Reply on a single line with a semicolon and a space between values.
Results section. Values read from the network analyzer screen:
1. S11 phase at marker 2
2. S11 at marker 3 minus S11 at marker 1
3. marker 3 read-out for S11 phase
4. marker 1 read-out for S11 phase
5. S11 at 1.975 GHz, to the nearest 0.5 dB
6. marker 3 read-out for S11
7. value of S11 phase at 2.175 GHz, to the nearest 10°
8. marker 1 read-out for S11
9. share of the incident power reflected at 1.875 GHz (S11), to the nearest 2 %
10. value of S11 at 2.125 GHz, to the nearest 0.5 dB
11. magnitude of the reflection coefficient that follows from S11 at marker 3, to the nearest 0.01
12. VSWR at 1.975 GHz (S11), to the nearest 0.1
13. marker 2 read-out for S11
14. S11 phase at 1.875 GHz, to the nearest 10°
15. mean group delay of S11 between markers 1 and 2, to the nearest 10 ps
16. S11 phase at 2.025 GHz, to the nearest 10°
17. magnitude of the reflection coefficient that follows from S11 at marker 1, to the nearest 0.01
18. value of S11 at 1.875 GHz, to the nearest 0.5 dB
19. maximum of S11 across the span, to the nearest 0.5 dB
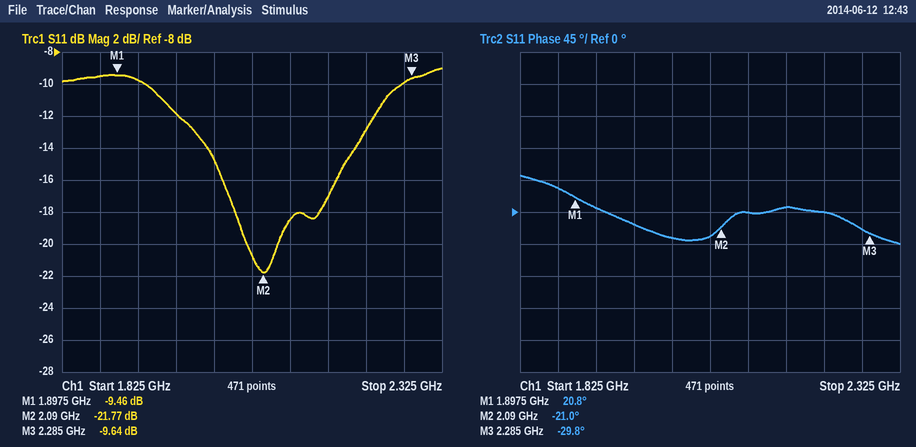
-21.0°; -0.18 dB; -29.8°; 20.8°; -12.0 dB; -9.64 dB; 10°; -9.46 dB; 12 %; -18.5 dB; 0.33; 1.7; -21.77 dB; 30°; 600 ps; -40°; 0.34; -9.5 dB; -9.0 dB
